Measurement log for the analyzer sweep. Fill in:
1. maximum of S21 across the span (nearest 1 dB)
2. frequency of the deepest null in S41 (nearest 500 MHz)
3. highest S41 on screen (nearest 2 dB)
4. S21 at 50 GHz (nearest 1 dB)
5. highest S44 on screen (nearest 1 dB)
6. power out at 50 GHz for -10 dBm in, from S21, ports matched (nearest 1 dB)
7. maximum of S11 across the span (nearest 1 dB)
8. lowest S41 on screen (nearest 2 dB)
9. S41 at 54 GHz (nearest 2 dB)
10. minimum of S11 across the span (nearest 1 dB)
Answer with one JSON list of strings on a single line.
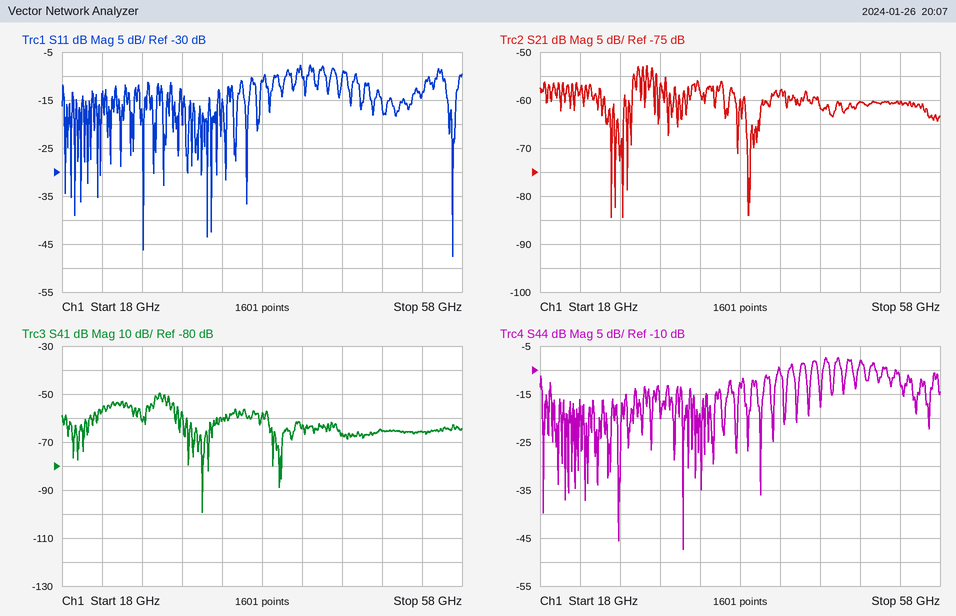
["-53 dB", "32.0 GHz", "-50 dB", "-60 dB", "-7 dB", "-70 dBm", "-8 dB", "-100 dB", "-66 dB", "-48 dB"]
